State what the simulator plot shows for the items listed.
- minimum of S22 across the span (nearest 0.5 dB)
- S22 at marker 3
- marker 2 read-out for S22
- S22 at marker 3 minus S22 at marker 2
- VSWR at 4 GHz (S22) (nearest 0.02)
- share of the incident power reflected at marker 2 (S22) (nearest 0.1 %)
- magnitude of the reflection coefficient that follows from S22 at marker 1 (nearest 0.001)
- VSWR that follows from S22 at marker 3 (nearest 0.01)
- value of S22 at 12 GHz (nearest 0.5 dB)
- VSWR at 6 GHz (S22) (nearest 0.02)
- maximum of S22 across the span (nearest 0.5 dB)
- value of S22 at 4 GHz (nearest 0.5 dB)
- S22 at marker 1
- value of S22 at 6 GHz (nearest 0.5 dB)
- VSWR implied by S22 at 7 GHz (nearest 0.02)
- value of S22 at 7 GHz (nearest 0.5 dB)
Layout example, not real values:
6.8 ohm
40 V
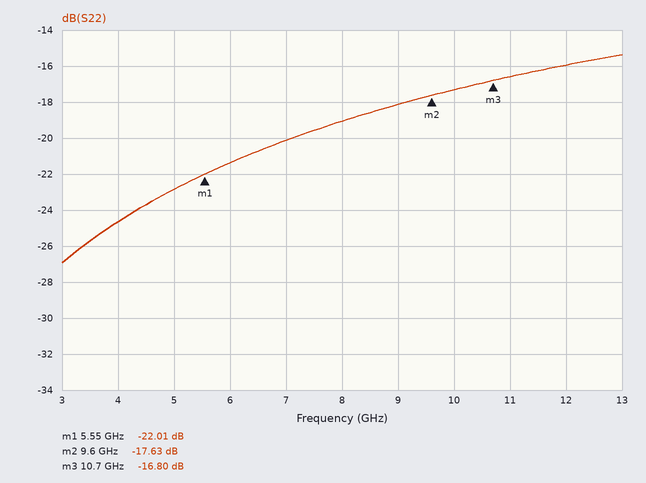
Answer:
-27.0 dB
-16.80 dB
-17.63 dB
0.83 dB
1.12
1.7 %
0.079
1.34
-16.0 dB
1.18
-15.5 dB
-24.5 dB
-22.01 dB
-21.5 dB
1.22
-20.0 dB
